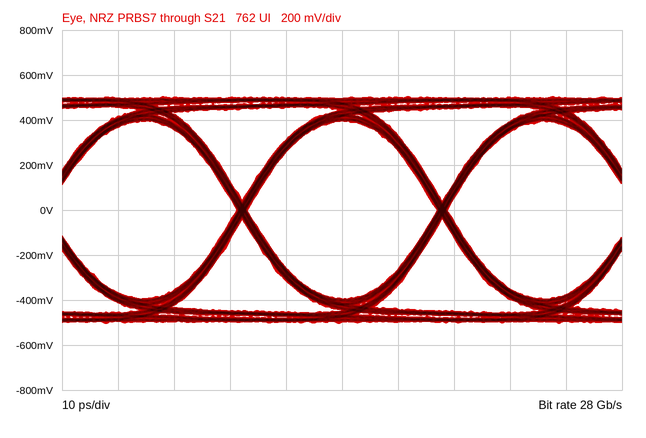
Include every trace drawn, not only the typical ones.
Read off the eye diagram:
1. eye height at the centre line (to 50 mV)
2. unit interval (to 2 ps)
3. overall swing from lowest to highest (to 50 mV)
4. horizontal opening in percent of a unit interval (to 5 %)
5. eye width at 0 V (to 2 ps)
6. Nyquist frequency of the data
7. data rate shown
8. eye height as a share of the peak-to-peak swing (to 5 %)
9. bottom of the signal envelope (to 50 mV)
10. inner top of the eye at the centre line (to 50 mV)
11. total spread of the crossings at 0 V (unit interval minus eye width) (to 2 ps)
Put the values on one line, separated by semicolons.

800 mV; 36 ps; 1.00 V; 95 %; 34 ps; 14 GHz; 28 Gb/s; 80 %; -500 mV; 400 mV; 2 ps
